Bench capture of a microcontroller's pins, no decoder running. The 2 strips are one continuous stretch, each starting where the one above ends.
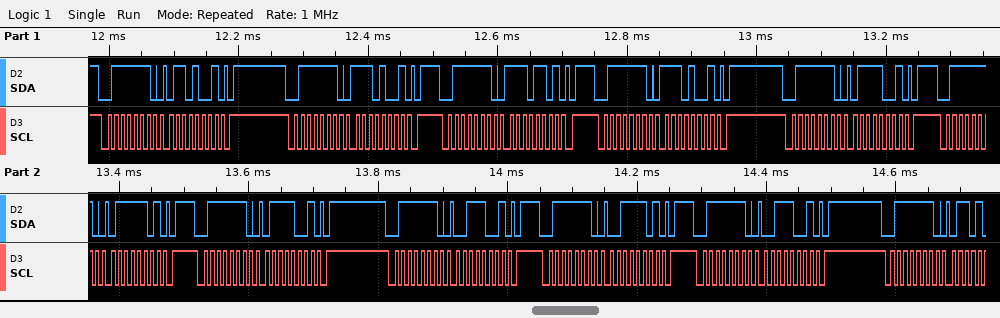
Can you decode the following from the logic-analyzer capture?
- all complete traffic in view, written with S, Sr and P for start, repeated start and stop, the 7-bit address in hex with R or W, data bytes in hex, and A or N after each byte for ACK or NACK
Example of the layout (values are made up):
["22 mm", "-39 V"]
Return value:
["S 3FW A 69 A P S 3FW A E9 A P S 3FW A ED A P S 3FW A E9 A P S 3FW A 79 A P S 3FW A 7D A P S 3FW A 79 A P S 3FW A 39 A P S 3FW A 3D A P S 3FW A 39 A P S 3FW A"]
